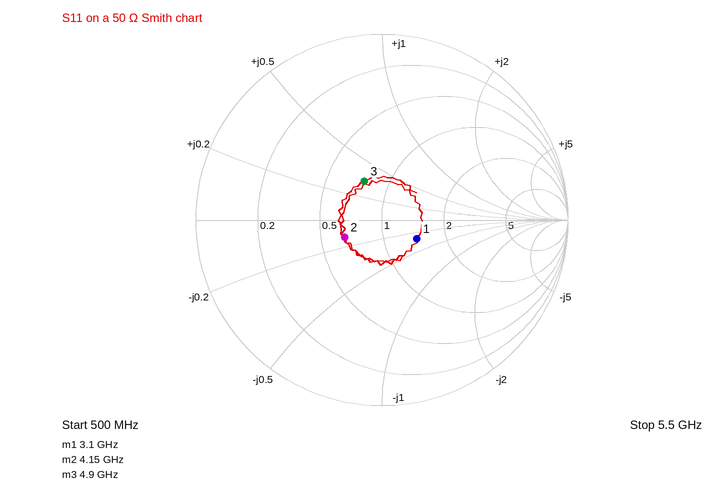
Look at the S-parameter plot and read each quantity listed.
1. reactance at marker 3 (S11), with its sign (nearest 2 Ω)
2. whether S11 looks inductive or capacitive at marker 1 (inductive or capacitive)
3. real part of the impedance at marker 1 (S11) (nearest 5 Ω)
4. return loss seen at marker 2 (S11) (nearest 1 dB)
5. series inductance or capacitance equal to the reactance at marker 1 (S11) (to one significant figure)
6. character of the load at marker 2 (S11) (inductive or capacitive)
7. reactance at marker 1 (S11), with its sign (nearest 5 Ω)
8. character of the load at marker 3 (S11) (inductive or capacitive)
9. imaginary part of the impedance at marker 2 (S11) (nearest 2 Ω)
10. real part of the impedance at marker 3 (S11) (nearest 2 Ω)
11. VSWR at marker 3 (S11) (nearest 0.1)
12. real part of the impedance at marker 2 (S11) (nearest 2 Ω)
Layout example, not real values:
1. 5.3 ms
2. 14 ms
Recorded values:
1. +16 Ω
2. capacitive
3. 70 Ω
4. 13 dB
5. 3 pF
6. capacitive
7. -15 Ω
8. inductive
9. -6 Ω
10. 38 Ω
11. 1.6
12. 32 Ω
